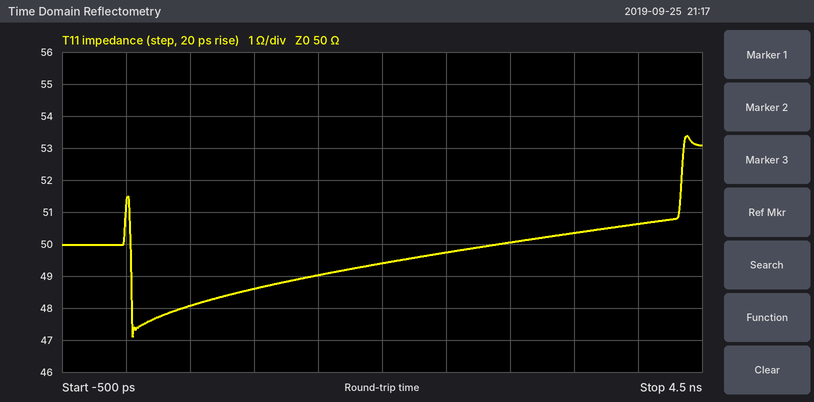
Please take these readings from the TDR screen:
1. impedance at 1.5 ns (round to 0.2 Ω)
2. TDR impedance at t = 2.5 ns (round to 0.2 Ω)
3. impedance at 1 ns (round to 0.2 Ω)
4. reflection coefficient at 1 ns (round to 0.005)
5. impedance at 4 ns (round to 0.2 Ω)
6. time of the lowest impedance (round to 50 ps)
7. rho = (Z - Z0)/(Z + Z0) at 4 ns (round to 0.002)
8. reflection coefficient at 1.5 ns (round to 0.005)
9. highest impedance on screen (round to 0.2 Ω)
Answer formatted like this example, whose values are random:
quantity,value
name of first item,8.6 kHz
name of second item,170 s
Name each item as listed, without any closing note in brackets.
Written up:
quantity,value
impedance at 1.5 ns,49.0 Ω
TDR impedance at t = 2.5 ns,49.8 Ω
impedance at 1 ns,48.6 Ω
reflection coefficient at 1 ns,-0.015
impedance at 4 ns,50.6 Ω
time of the lowest impedance,50 ps
rho = (Z - Z0)/(Z + Z0) at 4 ns,+0.006
reflection coefficient at 1.5 ns,-0.010
highest impedance on screen,53.4 Ω
